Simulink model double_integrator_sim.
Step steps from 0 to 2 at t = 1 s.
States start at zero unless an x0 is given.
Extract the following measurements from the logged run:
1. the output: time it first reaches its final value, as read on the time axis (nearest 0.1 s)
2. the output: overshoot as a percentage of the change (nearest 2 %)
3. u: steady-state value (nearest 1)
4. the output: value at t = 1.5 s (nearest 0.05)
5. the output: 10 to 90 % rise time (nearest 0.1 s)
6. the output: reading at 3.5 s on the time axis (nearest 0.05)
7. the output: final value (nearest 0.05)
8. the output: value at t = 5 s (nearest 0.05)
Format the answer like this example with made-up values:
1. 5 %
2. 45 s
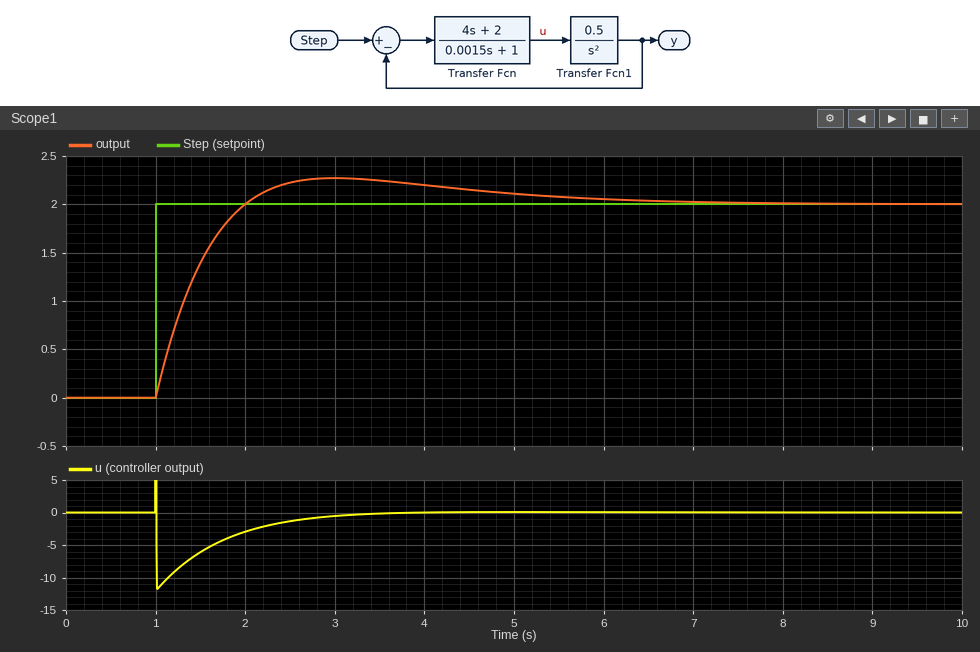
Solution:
1. 2.0 s
2. 14 %
3. 0
4. 1.40
5. 0.7 s
6. 2.25
7. 2.00
8. 2.10
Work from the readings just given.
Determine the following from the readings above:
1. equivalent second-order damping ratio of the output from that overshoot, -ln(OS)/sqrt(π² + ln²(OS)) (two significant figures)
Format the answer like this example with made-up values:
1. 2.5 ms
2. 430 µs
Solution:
1. 0.53
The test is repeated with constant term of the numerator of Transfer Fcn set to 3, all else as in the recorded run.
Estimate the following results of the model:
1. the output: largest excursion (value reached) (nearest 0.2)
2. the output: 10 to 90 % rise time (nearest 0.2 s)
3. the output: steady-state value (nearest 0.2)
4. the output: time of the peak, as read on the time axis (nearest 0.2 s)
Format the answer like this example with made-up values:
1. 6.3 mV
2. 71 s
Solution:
1. 2.4
2. 0.6 s
3. 2.0
4. 2.8 s
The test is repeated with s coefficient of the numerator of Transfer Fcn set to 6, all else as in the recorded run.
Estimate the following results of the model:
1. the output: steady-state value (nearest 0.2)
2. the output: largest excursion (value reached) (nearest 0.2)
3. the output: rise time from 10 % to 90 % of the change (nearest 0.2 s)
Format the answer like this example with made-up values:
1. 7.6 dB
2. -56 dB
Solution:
1. 2.0
2. 2.2
3. 0.6 s
